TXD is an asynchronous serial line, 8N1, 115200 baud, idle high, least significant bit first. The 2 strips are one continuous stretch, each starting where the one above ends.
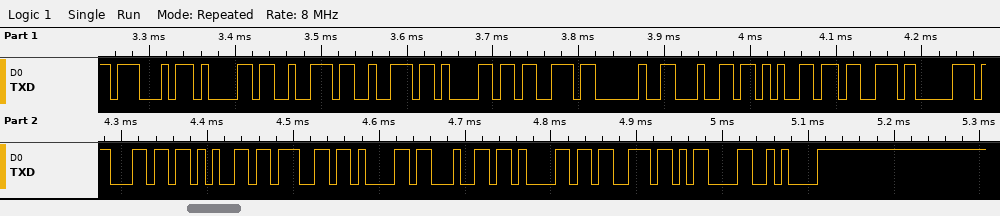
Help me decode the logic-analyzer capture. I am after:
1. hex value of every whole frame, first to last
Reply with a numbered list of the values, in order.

1. 47 61 72 72 61 73 20 64 65 73 70 6C 65 67 61 64 61 73 0D 0A
